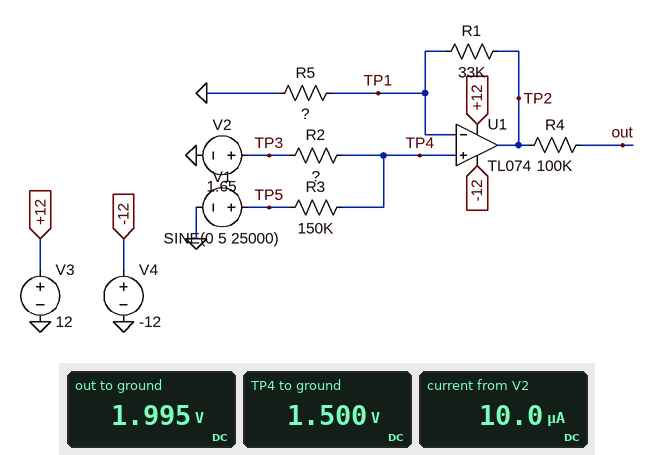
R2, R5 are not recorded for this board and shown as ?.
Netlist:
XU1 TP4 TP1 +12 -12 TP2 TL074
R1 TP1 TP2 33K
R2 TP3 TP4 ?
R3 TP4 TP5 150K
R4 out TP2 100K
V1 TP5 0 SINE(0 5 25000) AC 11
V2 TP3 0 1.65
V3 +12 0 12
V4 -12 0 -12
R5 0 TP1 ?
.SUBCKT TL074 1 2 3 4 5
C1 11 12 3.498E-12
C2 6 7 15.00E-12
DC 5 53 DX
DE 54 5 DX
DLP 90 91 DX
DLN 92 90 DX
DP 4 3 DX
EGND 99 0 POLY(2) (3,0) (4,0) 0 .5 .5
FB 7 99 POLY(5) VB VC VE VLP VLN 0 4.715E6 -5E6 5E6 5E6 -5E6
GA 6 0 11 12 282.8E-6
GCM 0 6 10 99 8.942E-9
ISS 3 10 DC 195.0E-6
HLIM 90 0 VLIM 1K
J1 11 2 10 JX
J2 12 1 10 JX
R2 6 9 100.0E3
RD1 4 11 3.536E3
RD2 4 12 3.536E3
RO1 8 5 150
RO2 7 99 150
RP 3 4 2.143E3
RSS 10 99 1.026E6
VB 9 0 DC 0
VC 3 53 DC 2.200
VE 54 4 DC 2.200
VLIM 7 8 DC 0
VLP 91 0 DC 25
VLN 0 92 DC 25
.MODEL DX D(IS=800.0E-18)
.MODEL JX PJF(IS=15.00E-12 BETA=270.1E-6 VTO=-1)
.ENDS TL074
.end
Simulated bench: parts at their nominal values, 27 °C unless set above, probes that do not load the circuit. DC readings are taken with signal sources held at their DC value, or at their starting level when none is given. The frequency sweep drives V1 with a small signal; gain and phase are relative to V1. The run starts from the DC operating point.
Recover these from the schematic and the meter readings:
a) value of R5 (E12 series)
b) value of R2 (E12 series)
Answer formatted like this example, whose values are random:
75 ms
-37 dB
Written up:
100 kΩ
15 kΩ
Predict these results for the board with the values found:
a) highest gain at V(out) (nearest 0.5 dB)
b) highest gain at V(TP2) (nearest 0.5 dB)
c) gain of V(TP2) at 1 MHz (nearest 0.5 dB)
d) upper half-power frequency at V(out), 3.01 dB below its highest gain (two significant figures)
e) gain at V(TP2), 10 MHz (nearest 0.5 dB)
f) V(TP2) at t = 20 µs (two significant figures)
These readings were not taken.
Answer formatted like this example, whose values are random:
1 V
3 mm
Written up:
-18.5 dB
-18.5 dB
-18.5 dB
3.6 MHz
-34.5 dB
2.0 V
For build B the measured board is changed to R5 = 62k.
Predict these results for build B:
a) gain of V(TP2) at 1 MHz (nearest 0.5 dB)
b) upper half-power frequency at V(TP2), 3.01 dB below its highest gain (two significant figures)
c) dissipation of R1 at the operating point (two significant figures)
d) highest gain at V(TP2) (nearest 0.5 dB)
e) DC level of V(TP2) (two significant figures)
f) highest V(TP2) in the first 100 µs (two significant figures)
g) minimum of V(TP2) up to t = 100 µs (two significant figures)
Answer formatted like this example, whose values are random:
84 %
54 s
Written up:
-17.5 dB
3.1 MHz
19 µW
-17.0 dB
2.3 V
3.0 V
1.6 V
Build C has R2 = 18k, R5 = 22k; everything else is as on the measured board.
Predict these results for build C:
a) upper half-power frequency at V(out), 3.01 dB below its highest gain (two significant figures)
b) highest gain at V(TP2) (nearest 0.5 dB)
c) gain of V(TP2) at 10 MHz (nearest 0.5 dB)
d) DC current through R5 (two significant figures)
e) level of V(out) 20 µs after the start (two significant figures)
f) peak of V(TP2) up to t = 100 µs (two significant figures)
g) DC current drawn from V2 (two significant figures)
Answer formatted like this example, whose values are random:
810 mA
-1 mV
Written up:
1.7 MHz
-11.5 dB
-33.5 dB
67 µA
3.7 V
5.0 V
9.8 µA
